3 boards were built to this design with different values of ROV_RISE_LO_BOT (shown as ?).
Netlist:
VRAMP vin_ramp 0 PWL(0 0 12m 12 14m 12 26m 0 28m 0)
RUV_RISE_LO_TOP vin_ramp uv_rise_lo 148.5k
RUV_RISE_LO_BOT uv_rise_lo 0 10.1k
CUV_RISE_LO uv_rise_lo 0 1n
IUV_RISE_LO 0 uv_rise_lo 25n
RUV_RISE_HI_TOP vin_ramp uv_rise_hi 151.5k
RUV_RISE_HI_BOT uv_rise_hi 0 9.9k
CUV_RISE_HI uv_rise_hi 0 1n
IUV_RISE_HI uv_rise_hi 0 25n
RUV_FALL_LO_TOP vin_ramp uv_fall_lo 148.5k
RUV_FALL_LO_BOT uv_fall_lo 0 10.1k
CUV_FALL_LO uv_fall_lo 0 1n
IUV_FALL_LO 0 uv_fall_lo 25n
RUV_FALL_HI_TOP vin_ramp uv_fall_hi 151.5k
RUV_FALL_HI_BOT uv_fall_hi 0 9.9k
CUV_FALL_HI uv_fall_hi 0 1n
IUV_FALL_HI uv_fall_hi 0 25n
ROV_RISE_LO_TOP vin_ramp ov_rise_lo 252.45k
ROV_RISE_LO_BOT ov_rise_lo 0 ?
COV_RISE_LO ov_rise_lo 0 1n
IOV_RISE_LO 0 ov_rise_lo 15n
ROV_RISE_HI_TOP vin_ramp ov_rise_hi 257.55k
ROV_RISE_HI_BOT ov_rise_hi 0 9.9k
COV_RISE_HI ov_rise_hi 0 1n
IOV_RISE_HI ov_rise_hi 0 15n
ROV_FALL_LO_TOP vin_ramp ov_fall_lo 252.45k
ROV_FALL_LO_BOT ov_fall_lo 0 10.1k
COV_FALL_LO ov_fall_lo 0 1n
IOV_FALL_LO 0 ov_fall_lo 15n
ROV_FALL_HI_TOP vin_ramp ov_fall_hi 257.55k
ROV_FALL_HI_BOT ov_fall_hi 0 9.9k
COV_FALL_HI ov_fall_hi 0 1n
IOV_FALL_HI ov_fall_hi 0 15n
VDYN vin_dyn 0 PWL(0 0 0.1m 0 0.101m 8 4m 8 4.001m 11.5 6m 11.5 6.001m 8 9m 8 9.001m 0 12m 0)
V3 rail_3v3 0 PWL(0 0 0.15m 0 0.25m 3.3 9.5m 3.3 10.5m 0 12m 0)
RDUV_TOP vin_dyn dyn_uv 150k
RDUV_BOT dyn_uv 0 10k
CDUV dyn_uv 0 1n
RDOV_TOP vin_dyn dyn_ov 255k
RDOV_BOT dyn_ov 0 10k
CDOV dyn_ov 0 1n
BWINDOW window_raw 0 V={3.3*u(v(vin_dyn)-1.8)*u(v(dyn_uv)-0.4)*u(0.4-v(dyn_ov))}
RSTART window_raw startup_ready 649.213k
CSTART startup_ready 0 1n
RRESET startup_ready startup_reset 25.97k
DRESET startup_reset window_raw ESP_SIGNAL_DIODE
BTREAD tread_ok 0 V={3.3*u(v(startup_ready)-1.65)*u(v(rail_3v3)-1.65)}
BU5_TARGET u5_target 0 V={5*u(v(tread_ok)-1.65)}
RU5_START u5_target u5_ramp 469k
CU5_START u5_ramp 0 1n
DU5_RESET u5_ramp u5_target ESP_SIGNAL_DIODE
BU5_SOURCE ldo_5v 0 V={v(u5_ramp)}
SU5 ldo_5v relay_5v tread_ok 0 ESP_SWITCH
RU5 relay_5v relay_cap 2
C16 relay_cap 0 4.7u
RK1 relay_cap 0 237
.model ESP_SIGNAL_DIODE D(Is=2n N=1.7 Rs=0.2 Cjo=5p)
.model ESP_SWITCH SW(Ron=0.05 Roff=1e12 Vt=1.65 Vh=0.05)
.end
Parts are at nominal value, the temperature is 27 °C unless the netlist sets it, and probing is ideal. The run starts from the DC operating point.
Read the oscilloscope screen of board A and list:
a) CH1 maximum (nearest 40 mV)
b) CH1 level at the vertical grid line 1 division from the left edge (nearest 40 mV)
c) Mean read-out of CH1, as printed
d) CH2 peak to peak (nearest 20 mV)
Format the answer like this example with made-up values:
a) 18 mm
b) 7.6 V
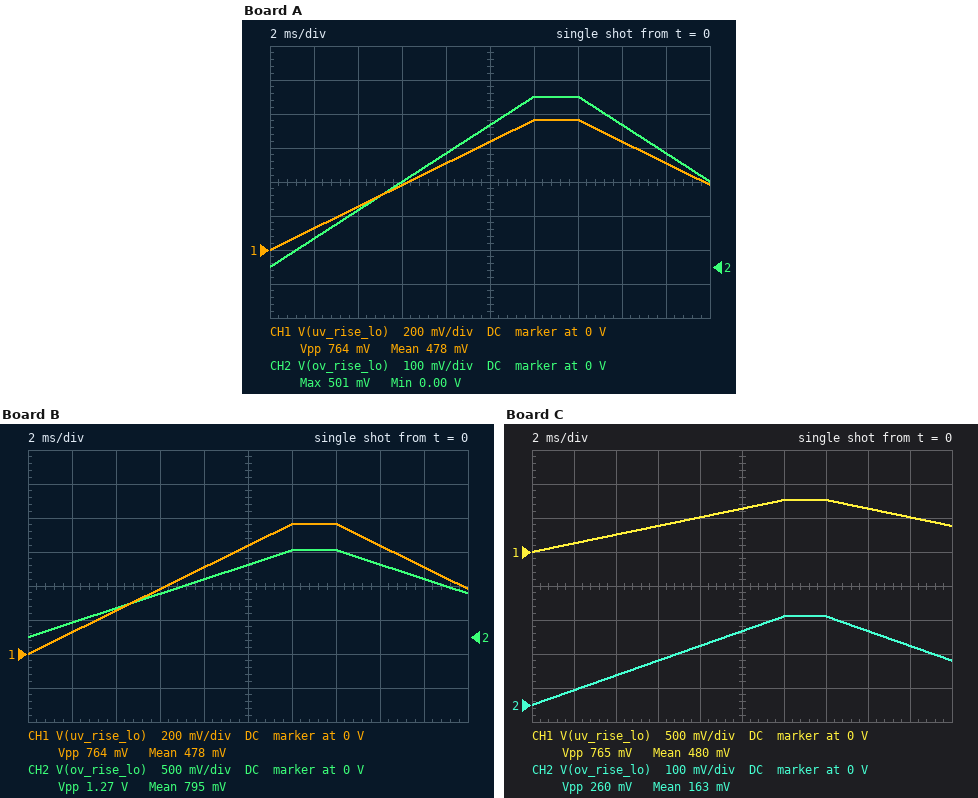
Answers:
a) 760 mV
b) 120 mV
c) 478 mV
d) 500 mV
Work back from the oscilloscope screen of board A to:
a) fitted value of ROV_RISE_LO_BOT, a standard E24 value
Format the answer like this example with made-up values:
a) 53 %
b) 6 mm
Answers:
a) 11 kΩ
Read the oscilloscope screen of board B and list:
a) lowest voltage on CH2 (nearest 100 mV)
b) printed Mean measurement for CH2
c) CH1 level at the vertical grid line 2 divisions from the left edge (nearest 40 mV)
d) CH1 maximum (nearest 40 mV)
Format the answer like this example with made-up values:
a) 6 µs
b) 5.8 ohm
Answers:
a) 0 V
b) 795 mV
c) 240 mV
d) 760 mV
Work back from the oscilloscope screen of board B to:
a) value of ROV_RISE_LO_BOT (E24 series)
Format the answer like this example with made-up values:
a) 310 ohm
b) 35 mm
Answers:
a) 30 kΩ
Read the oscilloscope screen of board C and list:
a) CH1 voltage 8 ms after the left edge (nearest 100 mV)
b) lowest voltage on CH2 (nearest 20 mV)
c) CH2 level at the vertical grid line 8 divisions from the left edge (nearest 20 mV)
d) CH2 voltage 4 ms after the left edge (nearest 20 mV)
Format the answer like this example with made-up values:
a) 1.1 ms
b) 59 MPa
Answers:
a) 500 mV
b) 0 V
c) 220 mV
d) 80 mV
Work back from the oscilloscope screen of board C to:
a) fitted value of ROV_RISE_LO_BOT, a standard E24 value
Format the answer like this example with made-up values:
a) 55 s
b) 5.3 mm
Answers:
a) 5.6 kΩ
